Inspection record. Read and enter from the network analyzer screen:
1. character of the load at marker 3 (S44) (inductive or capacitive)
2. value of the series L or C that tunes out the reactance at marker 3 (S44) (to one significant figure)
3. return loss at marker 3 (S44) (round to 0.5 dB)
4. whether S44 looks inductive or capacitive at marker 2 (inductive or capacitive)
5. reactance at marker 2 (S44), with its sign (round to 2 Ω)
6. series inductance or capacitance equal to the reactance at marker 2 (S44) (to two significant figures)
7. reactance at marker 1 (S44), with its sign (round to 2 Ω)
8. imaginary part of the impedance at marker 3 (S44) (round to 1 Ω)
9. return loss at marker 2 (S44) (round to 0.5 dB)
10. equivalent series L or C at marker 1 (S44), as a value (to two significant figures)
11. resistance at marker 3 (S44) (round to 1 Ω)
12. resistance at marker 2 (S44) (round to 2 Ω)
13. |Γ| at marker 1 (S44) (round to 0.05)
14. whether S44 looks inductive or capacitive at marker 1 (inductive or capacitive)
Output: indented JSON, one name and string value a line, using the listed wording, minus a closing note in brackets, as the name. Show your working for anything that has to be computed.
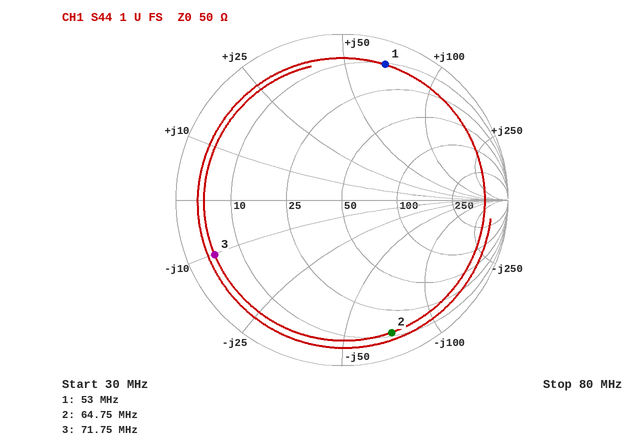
{
  "character of the load at marker 3 (S44)": "capacitive",
  "value of the series L or C that tunes out the reactance at marker 3 (S44)": "L = 10 Ω/(2π × 71.75 MHz) ≈ 22.2 nH, so 20 nH to one significant figure",
  "return loss at marker 3 (S44)": "1.5 dB",
  "whether S44 looks inductive or capacitive at marker 2": "capacitive",
  "reactance at marker 2 (S44), with its sign": "-70 Ω",
  "series inductance or capacitance equal to the reactance at marker 2 (S44)": "C = 1/(2π × 64.75 MHz × 70 Ω) ≈ 35 pF",
  "reactance at marker 1 (S44), with its sign": "+68 Ω",
  "imaginary part of the impedance at marker 3 (S44)": "-10 Ω",
  "return loss at marker 2 (S44)": "1.5 dB",
  "equivalent series L or C at marker 1 (S44), as a value": "L = 68 Ω/(2π × 53 MHz) ≈ 204 nH, so 200 nH to two significant figures",
  "resistance at marker 3 (S44)": "5 Ω",
  "resistance at marker 2 (S44)": "12 Ω",
  "|Γ| at marker 1 (S44)": "0.85",
  "whether S44 looks inductive or capacitive at marker 1": "inductive"
}
